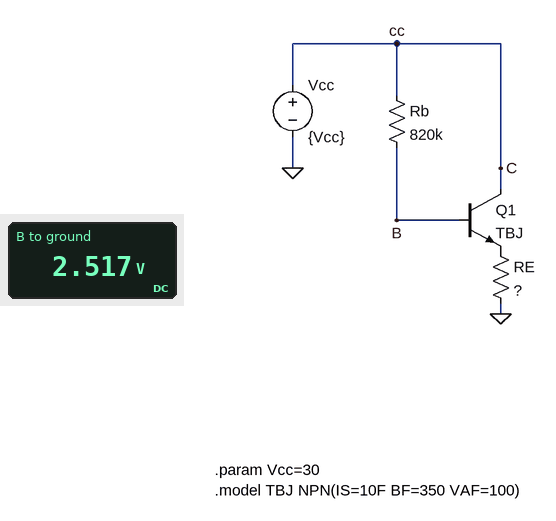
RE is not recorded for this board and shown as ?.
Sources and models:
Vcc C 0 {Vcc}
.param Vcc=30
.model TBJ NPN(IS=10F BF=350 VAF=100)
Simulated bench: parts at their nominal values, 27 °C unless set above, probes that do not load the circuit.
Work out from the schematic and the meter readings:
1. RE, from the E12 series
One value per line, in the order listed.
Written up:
120 Ω
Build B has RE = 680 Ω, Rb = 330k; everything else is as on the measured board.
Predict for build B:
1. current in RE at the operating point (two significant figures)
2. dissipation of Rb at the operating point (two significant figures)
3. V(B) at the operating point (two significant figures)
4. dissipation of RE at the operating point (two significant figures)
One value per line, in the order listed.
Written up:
20 mA
770 µW
14 V
260 mW
